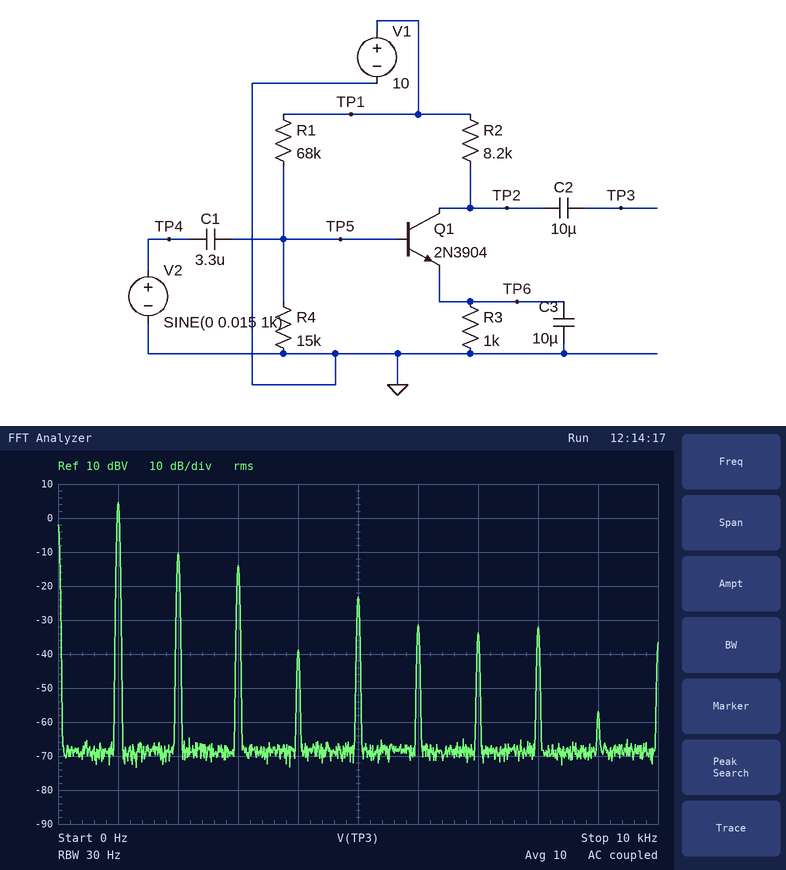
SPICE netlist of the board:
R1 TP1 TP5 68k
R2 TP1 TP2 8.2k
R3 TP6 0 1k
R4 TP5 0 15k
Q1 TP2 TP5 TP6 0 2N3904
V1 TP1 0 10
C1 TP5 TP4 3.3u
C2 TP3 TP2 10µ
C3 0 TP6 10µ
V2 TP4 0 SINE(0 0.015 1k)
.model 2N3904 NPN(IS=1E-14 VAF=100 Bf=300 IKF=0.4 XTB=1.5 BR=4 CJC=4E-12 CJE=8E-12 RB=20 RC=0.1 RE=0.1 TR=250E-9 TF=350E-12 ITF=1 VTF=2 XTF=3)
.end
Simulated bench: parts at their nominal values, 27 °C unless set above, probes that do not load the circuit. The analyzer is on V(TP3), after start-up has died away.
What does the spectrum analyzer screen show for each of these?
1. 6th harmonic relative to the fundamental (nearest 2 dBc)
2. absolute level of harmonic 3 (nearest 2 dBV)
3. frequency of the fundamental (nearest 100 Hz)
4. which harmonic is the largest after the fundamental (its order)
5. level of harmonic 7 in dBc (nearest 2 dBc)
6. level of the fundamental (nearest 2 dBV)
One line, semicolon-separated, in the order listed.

-36 dBc; -14 dBV; 1.0 kHz; 2; -38 dBc; 4 dBV
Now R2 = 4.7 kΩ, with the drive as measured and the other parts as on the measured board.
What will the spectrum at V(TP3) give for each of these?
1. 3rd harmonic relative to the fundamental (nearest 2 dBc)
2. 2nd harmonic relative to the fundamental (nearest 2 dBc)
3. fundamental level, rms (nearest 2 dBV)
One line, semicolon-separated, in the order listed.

-42 dBc; -20 dBc; 4 dBV
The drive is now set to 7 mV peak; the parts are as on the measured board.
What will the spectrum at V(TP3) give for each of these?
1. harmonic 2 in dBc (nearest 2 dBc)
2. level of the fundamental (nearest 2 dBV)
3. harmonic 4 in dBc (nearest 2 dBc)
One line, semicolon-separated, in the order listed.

-12 dBc; -2 dBV; -30 dBc
